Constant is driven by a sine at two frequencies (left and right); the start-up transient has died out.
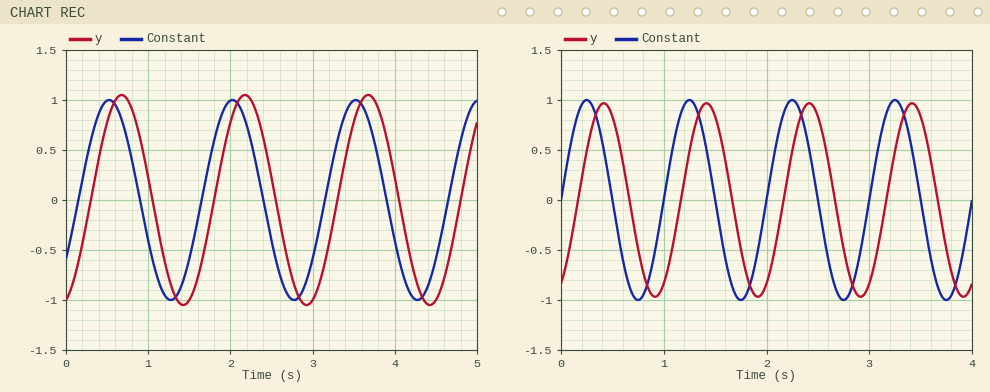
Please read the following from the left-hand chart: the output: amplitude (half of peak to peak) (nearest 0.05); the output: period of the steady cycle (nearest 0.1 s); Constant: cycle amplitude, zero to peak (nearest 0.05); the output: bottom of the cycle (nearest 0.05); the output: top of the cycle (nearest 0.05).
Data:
1.05
1.5 s
1.00
-1.05
1.05
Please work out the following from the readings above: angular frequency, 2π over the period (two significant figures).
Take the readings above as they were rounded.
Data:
4.2 rad/s
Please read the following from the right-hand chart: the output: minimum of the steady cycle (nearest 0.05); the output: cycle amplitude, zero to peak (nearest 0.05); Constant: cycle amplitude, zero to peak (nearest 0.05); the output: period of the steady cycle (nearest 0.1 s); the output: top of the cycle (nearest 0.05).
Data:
-0.95
0.95
1.00
1.0 s
0.95
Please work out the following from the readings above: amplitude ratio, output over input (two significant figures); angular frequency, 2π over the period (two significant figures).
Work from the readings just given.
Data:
0.95
6.3 rad/s
